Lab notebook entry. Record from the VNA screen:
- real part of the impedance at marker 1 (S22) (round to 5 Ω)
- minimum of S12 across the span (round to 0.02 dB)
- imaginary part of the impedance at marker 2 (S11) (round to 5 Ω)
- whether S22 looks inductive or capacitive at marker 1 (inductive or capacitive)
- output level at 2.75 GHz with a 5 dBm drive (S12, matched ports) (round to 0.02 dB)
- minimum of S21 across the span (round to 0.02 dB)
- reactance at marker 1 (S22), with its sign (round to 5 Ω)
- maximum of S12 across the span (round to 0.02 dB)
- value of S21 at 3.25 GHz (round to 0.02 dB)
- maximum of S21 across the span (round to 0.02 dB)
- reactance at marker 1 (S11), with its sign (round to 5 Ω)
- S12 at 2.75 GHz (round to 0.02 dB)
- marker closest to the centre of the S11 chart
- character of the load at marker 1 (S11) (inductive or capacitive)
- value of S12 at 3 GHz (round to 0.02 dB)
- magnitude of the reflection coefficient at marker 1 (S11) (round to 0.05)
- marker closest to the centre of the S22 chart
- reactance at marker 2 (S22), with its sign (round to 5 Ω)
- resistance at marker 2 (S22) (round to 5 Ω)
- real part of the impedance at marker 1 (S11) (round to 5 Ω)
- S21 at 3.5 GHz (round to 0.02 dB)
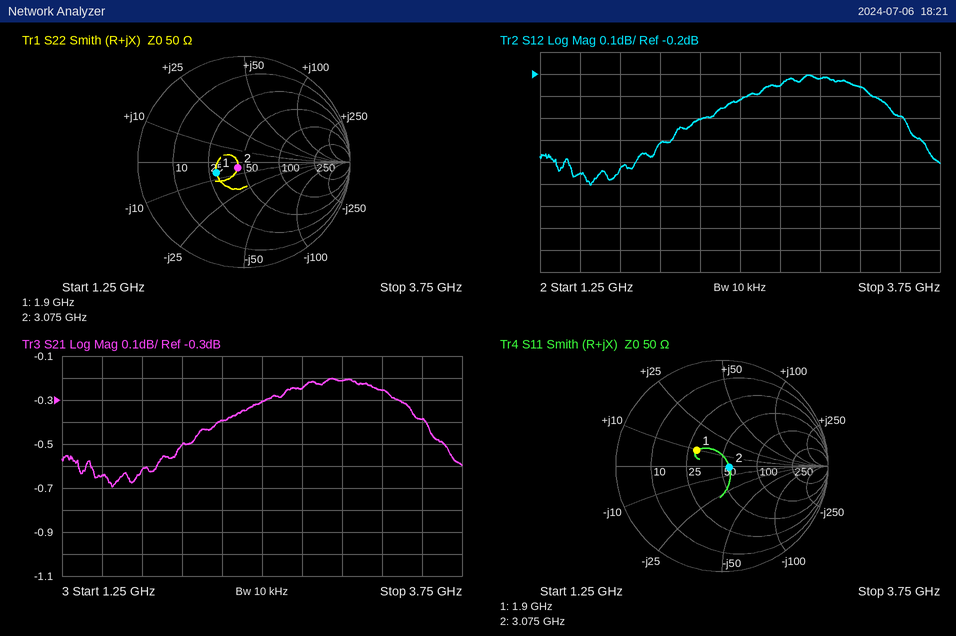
30 Ω
-0.70 dB
0 Ω
capacitive
4.74 dBm
-0.70 dB
-5 Ω
-0.20 dB
-0.26 dB
-0.20 dB
+10 Ω
-0.26 dB
marker 2
inductive
-0.22 dB
0.30
marker 2
-5 Ω
45 Ω
30 Ω
-0.38 dB
